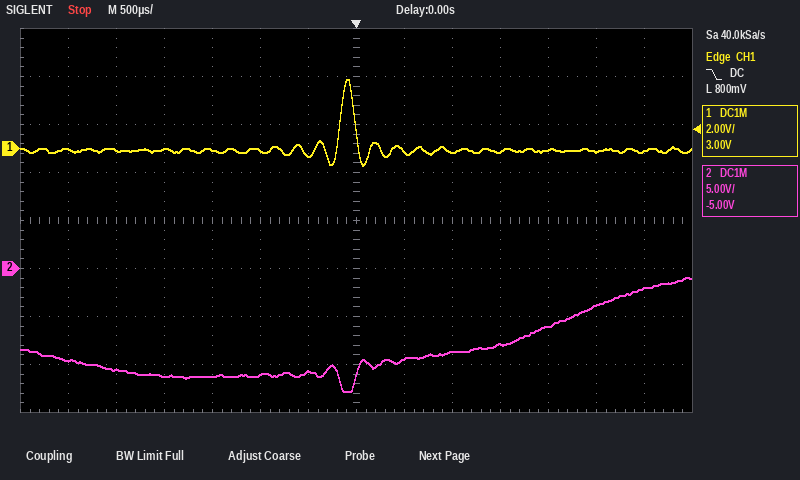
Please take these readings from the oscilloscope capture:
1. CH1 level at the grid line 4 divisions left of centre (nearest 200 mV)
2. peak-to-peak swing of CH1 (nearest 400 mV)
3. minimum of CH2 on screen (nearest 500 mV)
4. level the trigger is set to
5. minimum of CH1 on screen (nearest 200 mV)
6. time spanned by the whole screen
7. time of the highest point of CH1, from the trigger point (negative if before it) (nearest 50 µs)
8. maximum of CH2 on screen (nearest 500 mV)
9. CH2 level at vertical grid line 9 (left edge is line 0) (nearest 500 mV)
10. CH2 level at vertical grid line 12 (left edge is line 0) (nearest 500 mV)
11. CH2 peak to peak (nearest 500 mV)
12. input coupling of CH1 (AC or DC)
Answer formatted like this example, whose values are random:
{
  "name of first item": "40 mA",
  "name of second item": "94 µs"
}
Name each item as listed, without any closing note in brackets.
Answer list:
{
  "CH1 level at the grid line 4 divisions left of centre": "0.0 V",
  "peak-to-peak swing of CH1": "3.6 V",
  "minimum of CH2 on screen": "-13.0 V",
  "level the trigger is set to": "800 mV",
  "minimum of CH1 on screen": "-800 mV",
  "time spanned by the whole screen": "7 ms",
  "time of the highest point of CH1, from the trigger point (negative if before it)": "-100 µs",
  "maximum of CH2 on screen": "-1.0 V",
  "CH2 level at vertical grid line 9 (left edge is line 0)": "-8.5 V",
  "CH2 level at vertical grid line 12 (left edge is line 0)": "-4.0 V",
  "CH2 peak to peak": "12.0 V",
  "input coupling of CH1": "DC"
}
